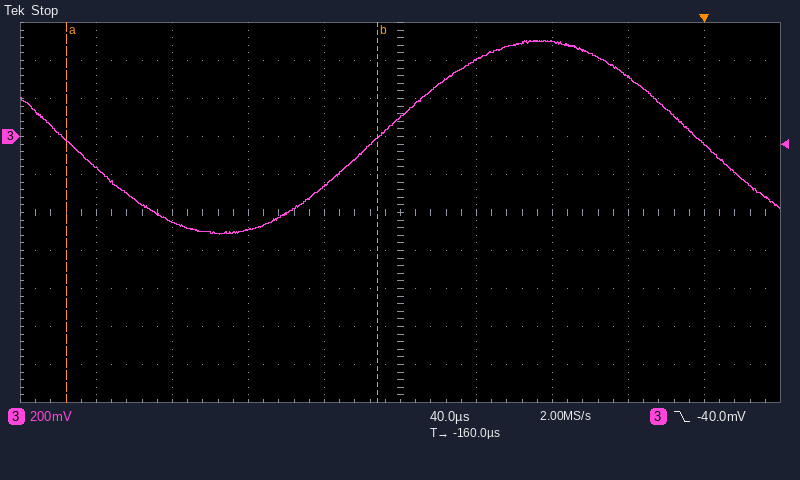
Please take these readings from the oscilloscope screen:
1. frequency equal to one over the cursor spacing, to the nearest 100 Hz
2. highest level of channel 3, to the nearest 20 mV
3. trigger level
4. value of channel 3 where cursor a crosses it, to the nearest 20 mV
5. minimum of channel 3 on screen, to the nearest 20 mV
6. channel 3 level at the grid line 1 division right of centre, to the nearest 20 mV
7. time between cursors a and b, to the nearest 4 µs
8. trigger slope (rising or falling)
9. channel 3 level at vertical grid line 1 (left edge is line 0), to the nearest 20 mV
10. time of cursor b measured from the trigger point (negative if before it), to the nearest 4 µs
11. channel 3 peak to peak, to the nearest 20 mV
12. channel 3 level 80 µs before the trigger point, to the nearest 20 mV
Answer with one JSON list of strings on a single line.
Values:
["6.1 kHz", "500 mV", "-40.0 mV", "-20 mV", "-520 mV", "400 mV", "164 µs", "falling", "-160 mV", "-172 µs", "1.02 V", "500 mV"]
